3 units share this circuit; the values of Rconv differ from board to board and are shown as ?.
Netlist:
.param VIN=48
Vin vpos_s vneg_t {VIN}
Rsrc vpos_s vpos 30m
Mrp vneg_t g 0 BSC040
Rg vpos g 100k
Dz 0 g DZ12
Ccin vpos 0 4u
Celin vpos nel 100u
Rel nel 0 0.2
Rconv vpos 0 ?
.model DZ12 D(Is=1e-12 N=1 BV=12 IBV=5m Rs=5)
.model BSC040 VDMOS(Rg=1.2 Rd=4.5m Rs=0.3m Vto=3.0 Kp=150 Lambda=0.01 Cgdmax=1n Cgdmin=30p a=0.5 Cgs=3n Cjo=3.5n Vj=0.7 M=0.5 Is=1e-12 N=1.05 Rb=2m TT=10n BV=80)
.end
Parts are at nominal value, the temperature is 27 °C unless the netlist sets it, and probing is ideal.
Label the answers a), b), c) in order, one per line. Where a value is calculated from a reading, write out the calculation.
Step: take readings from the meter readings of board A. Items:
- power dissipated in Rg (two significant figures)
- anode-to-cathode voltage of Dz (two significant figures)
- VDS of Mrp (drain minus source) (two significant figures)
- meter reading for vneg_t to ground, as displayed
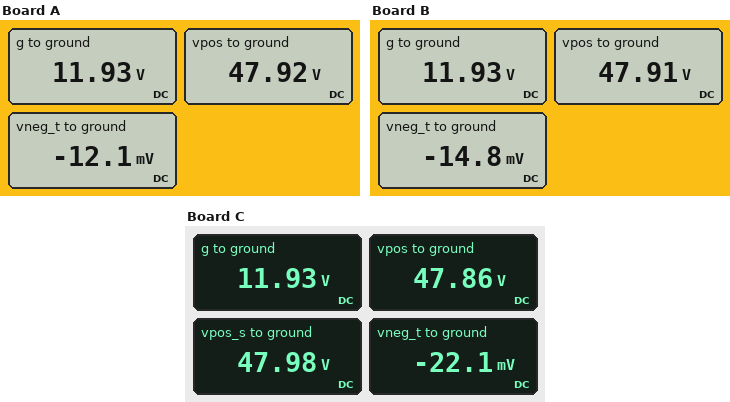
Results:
a) (47.92 V - 11.93 V)^2 / 100 kΩ = 13 mW
b) 0 V - 11.93 V = -12 V
c) -12.1 mV = -12 mV
d) -12.1 mV
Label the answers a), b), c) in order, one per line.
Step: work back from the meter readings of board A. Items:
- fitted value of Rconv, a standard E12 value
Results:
a) 22 Ω
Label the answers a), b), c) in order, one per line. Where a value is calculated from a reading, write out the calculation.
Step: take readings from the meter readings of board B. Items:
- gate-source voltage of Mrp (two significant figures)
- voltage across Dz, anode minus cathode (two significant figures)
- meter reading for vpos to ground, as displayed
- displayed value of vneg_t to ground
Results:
a) 11.93 V = 12 V
b) 0 V - 11.93 V = -12 V
c) 47.91 V
d) -14.8 mV
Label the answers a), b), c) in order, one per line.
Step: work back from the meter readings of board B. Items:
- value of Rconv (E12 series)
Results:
a) 18 Ω
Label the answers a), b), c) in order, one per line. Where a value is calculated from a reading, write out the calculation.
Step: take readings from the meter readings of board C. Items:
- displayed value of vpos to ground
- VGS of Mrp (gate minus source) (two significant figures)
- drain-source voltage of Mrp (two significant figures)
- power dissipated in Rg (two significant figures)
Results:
a) 47.86 V
b) 11.93 V = 12 V
c) -22.1 mV = -22 mV
d) (47.86 V - 11.93 V)^2 / 100 kΩ = 13 mW
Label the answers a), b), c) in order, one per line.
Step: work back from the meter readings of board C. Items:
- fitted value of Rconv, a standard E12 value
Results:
a) 12 Ω
